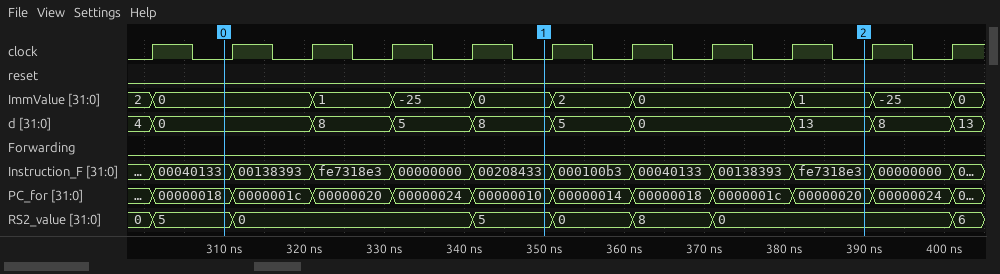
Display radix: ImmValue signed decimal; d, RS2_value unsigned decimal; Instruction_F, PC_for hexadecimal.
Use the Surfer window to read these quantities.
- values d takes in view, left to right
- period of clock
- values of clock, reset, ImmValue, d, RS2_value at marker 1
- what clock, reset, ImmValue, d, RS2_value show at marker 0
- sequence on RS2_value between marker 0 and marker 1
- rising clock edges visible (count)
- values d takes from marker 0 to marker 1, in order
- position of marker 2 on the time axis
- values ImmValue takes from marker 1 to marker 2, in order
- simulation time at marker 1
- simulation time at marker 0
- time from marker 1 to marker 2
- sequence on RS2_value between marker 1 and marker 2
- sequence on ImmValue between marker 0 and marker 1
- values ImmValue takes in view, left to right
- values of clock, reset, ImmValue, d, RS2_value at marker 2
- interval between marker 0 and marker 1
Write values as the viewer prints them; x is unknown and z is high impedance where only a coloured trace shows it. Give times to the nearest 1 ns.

4, 0, 8, 5, 8, 5, 0, 13, 8, 13
10 ns
clock=0, reset=0, ImmValue=0, d=8, RS2_value=5
clock=0, reset=0, ImmValue=0, d=0, RS2_value=5
5, 0, 5
11
0, 8, 5, 8
390 ns
0, 2, 0, 1
350 ns
310 ns
40 ns
5, 0, 8, 0
0, 1, -25, 0
2, 0, 1, -25, 0, 2, 0, 1, -25, 0
clock=0, reset=0, ImmValue=1, d=13, RS2_value=0
40 ns
